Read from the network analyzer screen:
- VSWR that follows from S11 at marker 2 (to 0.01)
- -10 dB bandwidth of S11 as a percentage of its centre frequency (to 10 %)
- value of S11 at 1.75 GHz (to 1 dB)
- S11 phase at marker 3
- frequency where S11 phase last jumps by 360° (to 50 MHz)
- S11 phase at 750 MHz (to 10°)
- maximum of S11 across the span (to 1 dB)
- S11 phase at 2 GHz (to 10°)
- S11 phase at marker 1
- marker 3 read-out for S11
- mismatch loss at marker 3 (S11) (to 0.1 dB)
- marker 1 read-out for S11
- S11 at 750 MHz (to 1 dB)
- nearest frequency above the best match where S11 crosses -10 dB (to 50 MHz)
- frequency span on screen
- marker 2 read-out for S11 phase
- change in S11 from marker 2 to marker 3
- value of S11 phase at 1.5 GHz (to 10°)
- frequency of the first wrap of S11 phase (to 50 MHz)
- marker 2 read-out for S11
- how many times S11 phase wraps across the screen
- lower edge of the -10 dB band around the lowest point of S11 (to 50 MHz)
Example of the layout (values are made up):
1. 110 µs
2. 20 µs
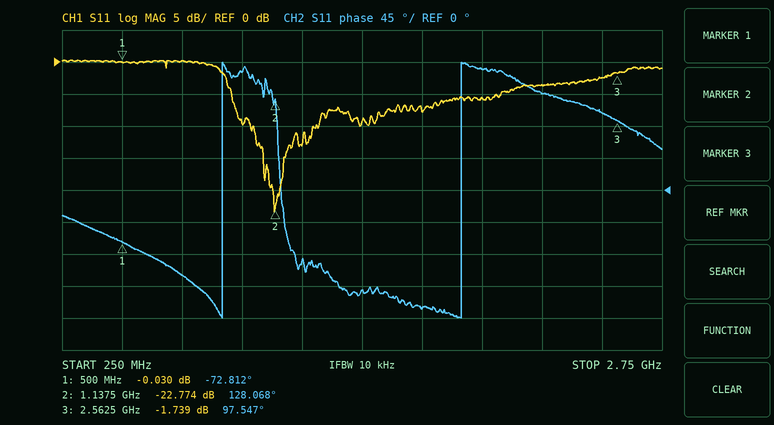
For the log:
1. 1.16
2. 20 %
3. -8 dB
4. 97.547°
5. 1.90 GHz
6. -120°
7. 0 dB
8. 170°
9. -72.812°
10. -1.739 dB
11. 4.8 dB
12. -0.030 dB
13. 0 dB
14. 1.30 GHz
15. 2.5 GHz
16. 128.068°
17. 21.035 dB
18. -140°
19. 900 MHz
20. -22.774 dB
21. 2
22. 1.05 GHz
